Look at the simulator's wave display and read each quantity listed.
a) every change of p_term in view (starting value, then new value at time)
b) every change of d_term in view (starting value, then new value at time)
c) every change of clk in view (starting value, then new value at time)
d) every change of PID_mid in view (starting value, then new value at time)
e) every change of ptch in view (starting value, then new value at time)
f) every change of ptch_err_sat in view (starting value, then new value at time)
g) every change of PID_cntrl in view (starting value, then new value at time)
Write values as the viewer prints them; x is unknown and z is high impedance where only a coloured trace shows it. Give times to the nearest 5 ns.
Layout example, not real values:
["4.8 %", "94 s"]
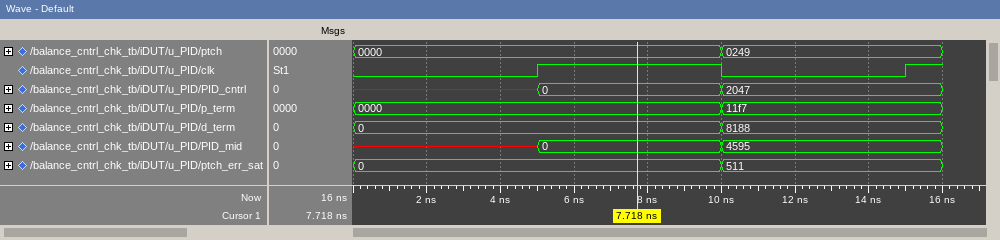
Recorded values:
["0000, 11f7 at 10 ns", "0, 8188 at 10 ns", "0, 1 at 5 ns, 0 at 10 ns, 1 at 15 ns", "x, 0 at 5 ns, 4595 at 10 ns", "0000, 0249 at 10 ns", "0, 511 at 10 ns", "x, 0 at 5 ns, 2047 at 10 ns"]
